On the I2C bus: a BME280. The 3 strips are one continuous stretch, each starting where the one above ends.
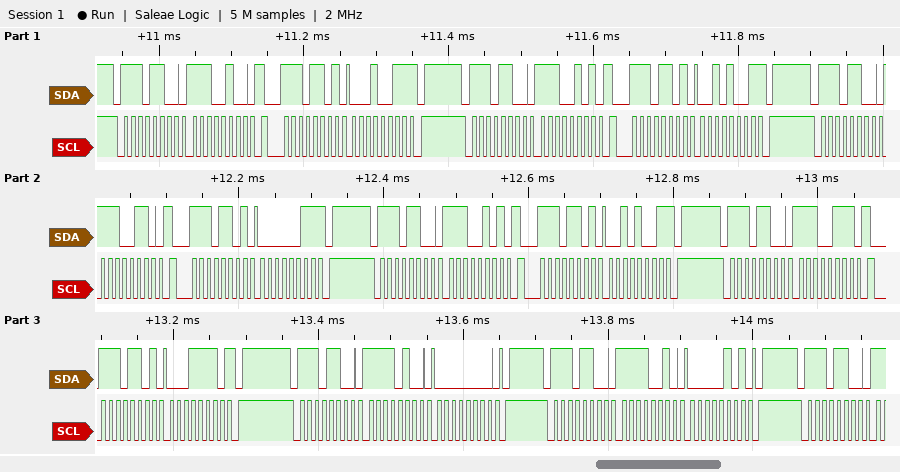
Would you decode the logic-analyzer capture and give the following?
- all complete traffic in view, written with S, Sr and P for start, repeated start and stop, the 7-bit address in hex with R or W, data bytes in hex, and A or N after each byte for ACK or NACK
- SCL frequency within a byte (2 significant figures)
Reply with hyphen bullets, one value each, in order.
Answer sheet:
- S 76W A E4 A Sr 76R A 13 N P S 76W A E5 A Sr 76R A 29 N P S 76W A E6 A Sr 76R A 03 N P S 76W A E5 A Sr 76R A 29 N P S 76W A E7 A Sr 76R A 1E N P S 76W A F4 A 00 A P S 76W A F2 A 05 A P S 76W A
- 100 kHz
